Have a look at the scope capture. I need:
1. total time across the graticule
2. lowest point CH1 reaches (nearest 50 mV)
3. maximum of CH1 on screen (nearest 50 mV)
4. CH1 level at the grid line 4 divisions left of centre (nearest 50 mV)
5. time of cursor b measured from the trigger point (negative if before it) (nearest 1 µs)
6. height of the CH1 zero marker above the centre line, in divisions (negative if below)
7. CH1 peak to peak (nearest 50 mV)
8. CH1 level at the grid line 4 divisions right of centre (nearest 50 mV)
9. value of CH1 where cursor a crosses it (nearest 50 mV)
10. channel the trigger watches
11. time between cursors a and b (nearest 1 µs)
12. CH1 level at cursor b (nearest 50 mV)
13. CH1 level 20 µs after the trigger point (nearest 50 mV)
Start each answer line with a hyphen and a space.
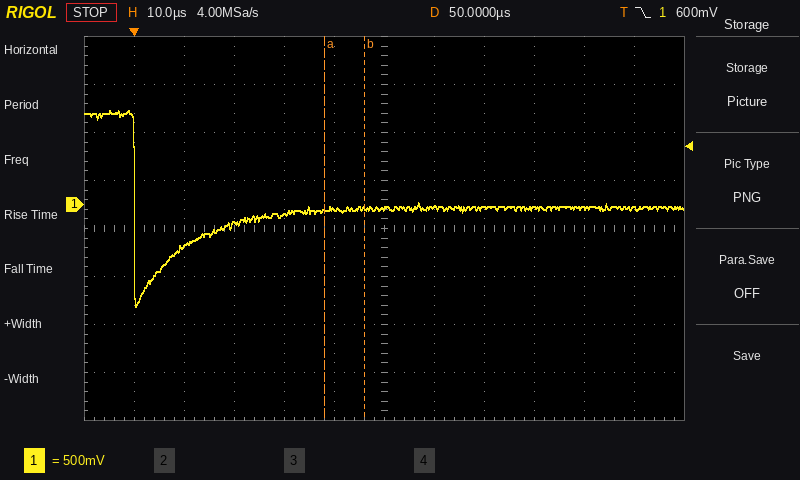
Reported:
- 120 µs
- -1.05 V
- 1.00 V
- -450 mV
- +46 µs
- +0.5 div
- 2.05 V
- -50 mV
- -50 mV
- CH1
- 8 µs
- -50 mV
- -200 mV
